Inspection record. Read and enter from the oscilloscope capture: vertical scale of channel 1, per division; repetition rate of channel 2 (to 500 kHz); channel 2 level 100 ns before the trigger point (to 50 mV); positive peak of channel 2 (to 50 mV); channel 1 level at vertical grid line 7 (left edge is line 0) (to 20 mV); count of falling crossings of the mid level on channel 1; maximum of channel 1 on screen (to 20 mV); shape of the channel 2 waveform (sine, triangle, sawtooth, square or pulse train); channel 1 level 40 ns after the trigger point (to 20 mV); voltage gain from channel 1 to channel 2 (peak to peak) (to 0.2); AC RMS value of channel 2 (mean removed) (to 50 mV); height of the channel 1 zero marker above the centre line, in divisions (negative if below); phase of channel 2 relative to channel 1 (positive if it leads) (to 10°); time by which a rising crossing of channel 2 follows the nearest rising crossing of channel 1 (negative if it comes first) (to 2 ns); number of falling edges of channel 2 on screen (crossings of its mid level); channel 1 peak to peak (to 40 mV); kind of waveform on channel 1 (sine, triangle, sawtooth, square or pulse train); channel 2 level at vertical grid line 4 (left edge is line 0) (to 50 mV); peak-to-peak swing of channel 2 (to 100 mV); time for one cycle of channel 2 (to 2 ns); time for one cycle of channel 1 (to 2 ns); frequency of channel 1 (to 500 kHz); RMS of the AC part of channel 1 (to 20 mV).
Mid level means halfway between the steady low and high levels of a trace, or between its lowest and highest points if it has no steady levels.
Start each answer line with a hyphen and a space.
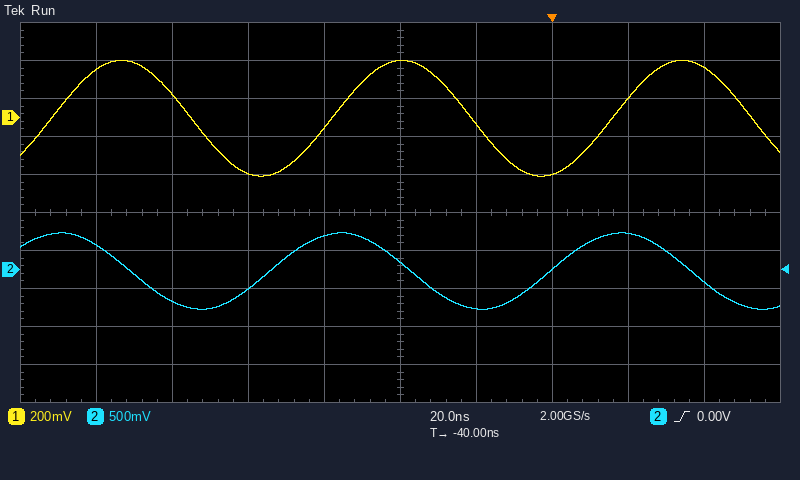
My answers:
- 200 mV
- 13.5 MHz
- -400 mV
- 500 mV
- -300 mV
- 3
- 300 mV
- sine
- 260 mV
- 1.6
- 350 mV
- +2.5 div
- +80°
- -16 ns
- 3
- 600 mV
- sine
- 450 mV
- 1.00 V
- 74 ns
- 74 ns
- 13.5 MHz
- 220 mV
